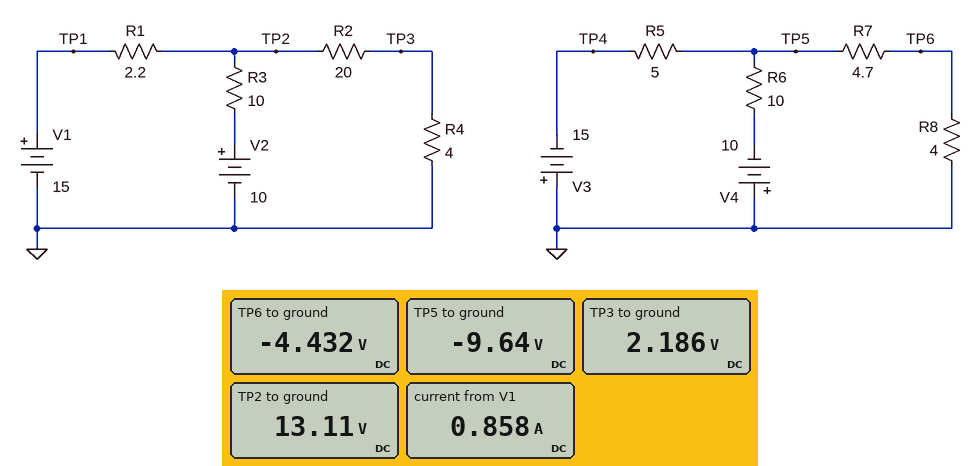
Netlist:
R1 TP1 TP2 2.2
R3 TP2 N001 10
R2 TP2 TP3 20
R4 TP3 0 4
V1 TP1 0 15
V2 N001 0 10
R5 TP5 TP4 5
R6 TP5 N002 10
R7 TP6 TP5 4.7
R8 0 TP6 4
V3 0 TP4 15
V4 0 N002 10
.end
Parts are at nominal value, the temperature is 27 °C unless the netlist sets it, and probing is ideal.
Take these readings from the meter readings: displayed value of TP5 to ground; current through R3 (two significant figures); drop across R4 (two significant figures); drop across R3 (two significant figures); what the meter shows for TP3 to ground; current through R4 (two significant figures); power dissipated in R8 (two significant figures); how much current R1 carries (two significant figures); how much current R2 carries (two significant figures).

-9.64 V
310 mA
2.2 V
3.1 V
2.186 V
550 mA
4.9 W
860 mA
550 mA
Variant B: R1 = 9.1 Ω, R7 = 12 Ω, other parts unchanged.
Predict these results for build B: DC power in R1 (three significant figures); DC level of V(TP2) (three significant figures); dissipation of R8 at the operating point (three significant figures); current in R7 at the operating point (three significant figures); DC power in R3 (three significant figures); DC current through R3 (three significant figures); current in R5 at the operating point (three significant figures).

2.20 W
10.5 V
1.90 W
690 mA
27.9 mW
52.8 mA
793 mA
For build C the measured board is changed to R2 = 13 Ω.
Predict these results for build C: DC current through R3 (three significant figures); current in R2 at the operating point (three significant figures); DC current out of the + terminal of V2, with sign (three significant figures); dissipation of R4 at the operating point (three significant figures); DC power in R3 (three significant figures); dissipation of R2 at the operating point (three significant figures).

275 mA
750 mA
-275 mA
2.25 W
754 mW
7.31 W
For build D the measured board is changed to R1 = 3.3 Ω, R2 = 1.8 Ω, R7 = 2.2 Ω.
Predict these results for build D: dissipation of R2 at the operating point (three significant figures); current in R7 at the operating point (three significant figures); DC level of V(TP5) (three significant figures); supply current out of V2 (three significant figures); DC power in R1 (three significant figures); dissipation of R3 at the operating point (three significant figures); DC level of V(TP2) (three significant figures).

4.97 W
1.40 A
-8.67 V
36.3 mA
8.72 W
13.2 mW
9.64 V
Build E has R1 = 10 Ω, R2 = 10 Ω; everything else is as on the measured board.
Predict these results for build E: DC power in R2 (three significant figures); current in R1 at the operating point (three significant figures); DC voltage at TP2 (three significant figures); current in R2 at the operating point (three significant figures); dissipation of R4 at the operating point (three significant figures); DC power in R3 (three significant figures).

4.33 W
579 mA
9.21 V
658 mA
1.73 W
62.3 mW
